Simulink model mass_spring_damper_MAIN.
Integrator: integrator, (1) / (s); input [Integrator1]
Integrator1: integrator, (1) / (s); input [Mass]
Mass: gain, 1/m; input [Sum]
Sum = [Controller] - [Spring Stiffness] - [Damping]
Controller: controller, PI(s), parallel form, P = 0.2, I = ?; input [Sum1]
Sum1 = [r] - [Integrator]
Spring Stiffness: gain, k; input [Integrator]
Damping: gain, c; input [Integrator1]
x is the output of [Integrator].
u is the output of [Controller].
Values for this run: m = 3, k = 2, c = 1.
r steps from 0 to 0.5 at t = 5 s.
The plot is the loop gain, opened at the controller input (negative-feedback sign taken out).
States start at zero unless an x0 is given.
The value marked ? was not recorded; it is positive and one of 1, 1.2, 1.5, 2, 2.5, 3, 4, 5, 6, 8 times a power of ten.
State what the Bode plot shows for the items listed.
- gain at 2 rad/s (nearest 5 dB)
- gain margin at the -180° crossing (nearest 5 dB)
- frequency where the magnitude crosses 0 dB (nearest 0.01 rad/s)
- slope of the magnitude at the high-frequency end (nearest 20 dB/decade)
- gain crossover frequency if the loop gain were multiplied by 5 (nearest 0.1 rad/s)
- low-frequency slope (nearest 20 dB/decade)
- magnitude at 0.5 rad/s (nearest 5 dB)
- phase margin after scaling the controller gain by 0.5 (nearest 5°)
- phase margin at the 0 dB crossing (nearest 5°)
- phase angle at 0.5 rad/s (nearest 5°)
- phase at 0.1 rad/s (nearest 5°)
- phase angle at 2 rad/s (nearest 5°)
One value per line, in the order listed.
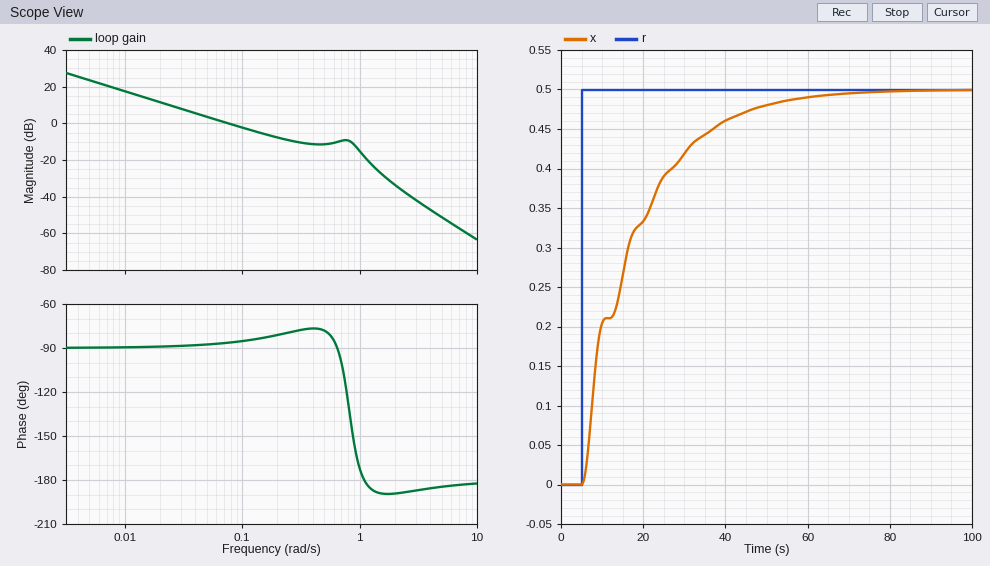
-35 dB
20 dB
0.08 rad/s
-40 dB/decade
1.0 rad/s
-20 dB/decade
-10 dB
90°
95°
-80°
-85°
-190°
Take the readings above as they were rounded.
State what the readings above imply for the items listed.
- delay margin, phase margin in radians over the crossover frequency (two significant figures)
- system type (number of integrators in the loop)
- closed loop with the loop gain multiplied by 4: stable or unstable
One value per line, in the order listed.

21 s
1
stable
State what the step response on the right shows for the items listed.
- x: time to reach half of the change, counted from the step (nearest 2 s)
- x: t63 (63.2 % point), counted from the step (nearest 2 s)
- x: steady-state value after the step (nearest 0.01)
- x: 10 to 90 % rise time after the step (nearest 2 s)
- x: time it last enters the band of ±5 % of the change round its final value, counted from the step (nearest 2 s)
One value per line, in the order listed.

10 s
12 s
0.50
30 s
42 s
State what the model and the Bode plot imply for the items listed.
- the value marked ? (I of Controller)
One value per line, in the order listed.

0.15
